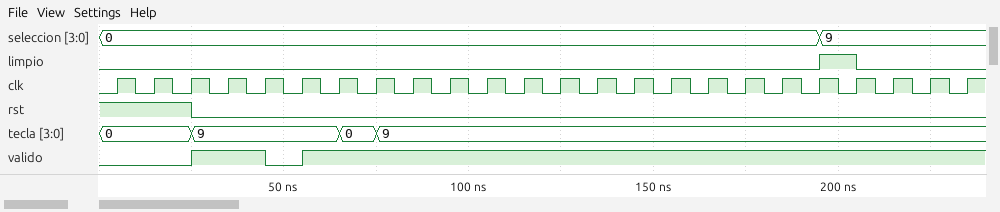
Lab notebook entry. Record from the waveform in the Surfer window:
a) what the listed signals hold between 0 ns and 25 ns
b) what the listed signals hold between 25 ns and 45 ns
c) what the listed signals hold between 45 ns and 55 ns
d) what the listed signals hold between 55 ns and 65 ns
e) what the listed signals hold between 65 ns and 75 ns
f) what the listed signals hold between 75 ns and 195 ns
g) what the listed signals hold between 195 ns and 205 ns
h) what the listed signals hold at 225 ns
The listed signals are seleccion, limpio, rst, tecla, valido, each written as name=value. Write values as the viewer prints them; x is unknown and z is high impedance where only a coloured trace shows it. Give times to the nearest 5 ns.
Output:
seleccion=0, limpio=0, rst=1, tecla=0, valido=0
seleccion=0, limpio=0, rst=0, tecla=9, valido=1
seleccion=0, limpio=0, rst=0, tecla=9, valido=0
seleccion=0, limpio=0, rst=0, tecla=9, valido=1
seleccion=0, limpio=0, rst=0, tecla=0, valido=1
seleccion=0, limpio=0, rst=0, tecla=9, valido=1
seleccion=9, limpio=1, rst=0, tecla=9, valido=1
seleccion=9, limpio=0, rst=0, tecla=9, valido=1
